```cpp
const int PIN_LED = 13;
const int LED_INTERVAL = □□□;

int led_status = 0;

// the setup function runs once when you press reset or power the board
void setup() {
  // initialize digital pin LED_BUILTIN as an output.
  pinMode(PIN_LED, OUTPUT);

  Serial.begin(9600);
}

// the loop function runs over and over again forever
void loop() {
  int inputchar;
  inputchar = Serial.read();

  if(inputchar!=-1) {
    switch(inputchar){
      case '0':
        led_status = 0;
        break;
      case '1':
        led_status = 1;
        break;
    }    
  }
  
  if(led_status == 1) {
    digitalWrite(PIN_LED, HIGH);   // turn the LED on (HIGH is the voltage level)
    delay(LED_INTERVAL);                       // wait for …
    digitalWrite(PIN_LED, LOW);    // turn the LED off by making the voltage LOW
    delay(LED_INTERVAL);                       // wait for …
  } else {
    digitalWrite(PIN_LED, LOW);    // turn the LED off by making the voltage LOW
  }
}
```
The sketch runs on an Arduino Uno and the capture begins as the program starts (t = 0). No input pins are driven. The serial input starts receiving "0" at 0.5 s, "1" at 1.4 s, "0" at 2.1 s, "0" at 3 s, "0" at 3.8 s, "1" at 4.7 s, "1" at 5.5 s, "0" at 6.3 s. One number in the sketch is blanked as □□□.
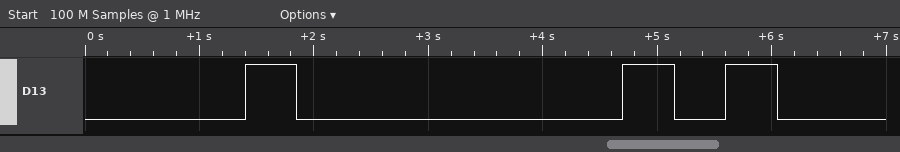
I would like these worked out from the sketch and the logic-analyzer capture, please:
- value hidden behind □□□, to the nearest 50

450
